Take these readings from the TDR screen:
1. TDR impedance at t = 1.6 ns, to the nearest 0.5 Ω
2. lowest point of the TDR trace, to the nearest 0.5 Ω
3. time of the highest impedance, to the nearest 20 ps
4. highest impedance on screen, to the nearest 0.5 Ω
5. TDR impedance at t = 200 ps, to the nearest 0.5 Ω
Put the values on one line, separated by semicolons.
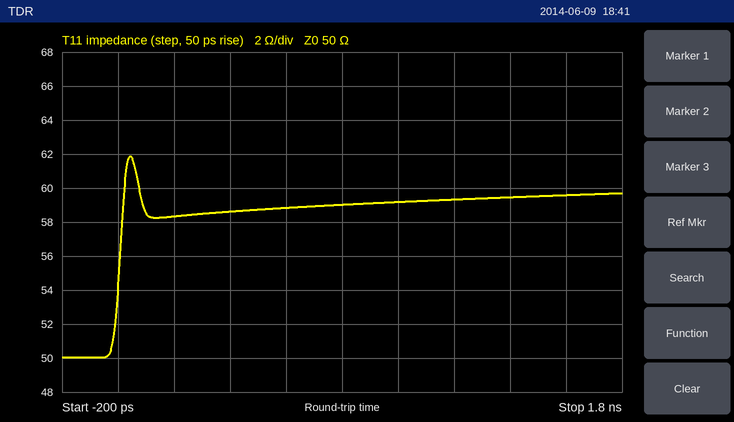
59.5 Ω; 50.0 Ω; 40 ps; 62.0 Ω; 58.5 Ω
